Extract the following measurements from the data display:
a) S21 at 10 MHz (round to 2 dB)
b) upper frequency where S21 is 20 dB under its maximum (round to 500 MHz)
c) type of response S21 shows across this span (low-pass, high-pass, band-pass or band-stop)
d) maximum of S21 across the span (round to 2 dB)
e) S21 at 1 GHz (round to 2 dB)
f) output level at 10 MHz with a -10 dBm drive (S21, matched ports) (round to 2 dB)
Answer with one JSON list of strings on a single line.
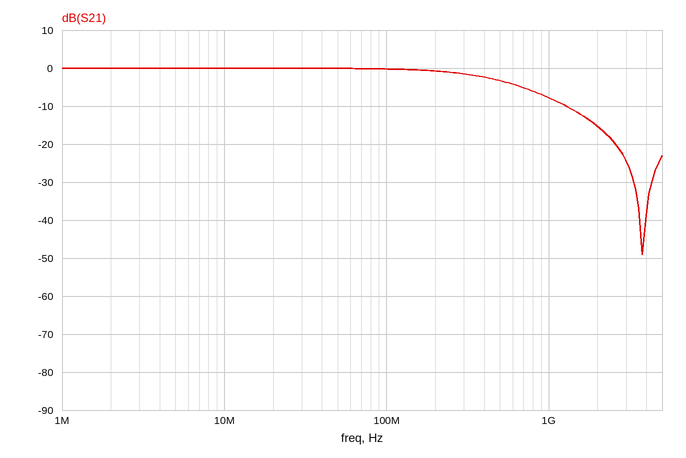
["0 dB", "2.5 GHz", "low-pass", "0 dB", "-8 dB", "-10 dBm"]
